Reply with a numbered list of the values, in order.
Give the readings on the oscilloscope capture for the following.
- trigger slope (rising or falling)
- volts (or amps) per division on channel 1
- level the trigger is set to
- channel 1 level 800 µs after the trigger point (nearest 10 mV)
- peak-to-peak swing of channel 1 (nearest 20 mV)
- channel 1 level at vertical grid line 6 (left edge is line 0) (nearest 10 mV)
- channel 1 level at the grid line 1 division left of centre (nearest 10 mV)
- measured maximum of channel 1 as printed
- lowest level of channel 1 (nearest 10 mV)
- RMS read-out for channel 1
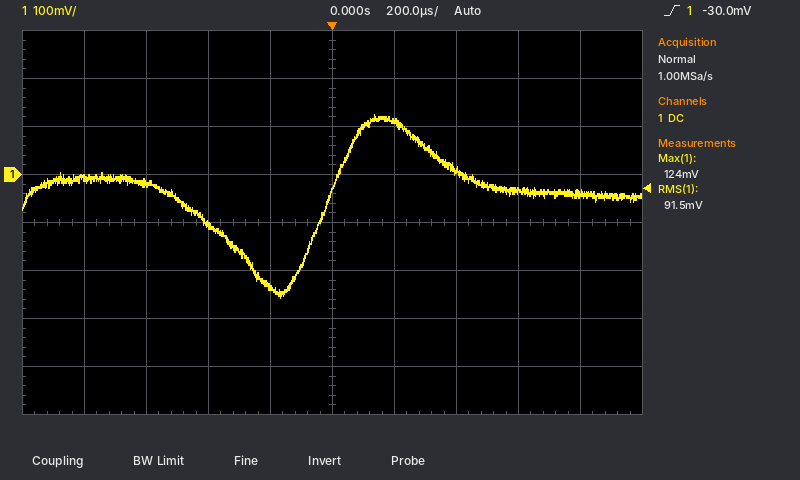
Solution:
1. rising
2. 100 mV
3. -30.0 mV
4. -40 mV
5. 380 mV
6. 110 mV
7. -230 mV
8. 124 mV
9. -260 mV
10. 91.5 mV
